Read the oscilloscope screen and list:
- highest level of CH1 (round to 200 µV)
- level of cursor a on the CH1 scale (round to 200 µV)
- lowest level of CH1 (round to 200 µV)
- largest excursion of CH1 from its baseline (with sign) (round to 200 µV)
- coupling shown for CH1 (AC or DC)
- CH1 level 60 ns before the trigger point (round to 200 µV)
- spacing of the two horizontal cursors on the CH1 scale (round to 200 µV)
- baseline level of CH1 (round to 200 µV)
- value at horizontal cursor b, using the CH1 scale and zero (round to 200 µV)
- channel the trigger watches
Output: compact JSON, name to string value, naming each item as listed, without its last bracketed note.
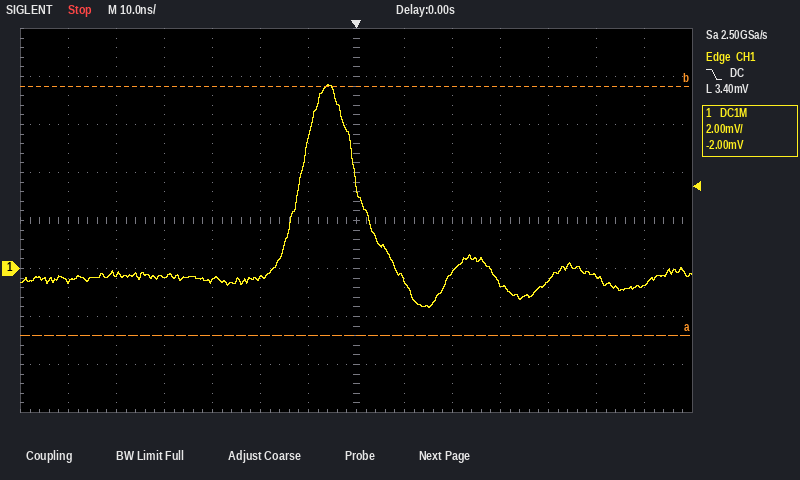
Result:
{"highest level of CH1": "7.6 mV", "level of cursor a on the CH1 scale": "-2.8 mV", "lowest level of CH1": "-1.6 mV", "largest excursion of CH1 from its baseline (with sign)": "+8.0 mV", "coupling shown for CH1": "DC", "CH1 level 60 ns before the trigger point": "-600 µV", "spacing of the two horizontal cursors on the CH1 scale": "10.4 mV", "baseline level of CH1": "-400 µV", "value at horizontal cursor b, using the CH1 scale and zero": "7.6 mV", "channel the trigger watches": "CH1"}
